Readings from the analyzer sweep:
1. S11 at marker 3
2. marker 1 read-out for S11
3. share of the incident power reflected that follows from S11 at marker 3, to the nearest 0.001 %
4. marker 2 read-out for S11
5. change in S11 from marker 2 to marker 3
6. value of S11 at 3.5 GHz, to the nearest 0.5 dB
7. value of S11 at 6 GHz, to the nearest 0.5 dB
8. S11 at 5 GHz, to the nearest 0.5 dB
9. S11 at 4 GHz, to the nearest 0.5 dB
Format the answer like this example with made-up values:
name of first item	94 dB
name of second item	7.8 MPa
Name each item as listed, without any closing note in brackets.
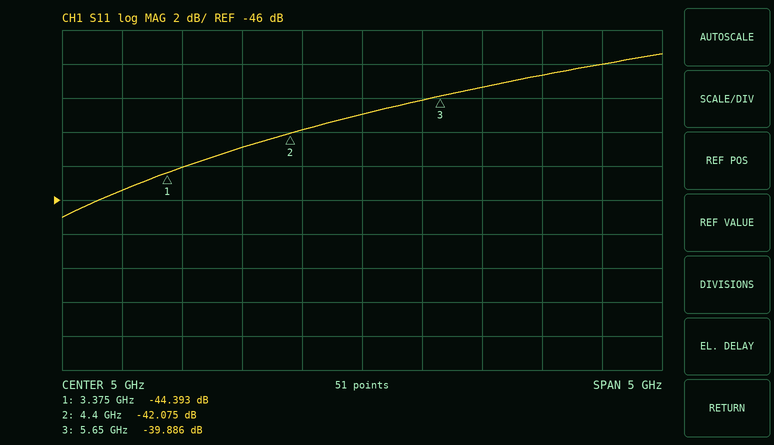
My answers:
S11 at marker 3	-39.886 dB
marker 1 read-out for S11	-44.393 dB
share of the incident power reflected that follows from S11 at marker 3, to the nearest 0.001 %	0.010 %
marker 2 read-out for S11	-42.075 dB
change in S11 from marker 2 to marker 3	2.189 dB
value of S11 at 3.5 GHz, to the nearest 0.5 dB	-44.0 dB
value of S11 at 6 GHz, to the nearest 0.5 dB	-39.5 dB
S11 at 5 GHz, to the nearest 0.5 dB	-41.0 dB
S11 at 4 GHz, to the nearest 0.5 dB	-43.0 dB
